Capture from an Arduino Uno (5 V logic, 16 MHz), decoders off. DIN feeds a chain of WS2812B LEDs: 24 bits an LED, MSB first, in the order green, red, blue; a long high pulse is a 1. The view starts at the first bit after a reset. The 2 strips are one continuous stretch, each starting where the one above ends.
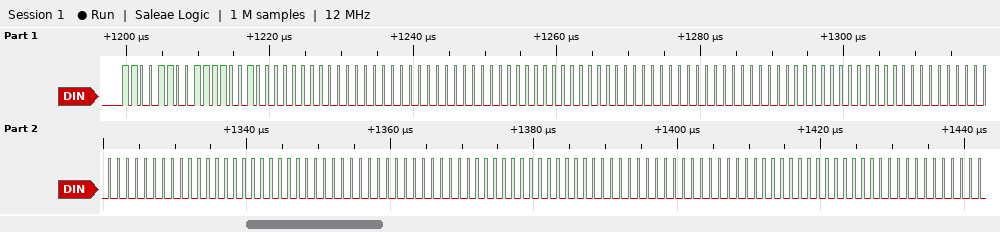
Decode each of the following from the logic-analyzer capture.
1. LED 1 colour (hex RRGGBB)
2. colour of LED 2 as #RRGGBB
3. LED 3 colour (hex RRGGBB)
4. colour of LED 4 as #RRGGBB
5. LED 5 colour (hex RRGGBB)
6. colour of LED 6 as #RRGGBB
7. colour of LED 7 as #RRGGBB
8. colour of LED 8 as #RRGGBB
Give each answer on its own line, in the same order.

#F2CC00
#000000
#000000
#000000
#000000
#000000
#000000
#000000
